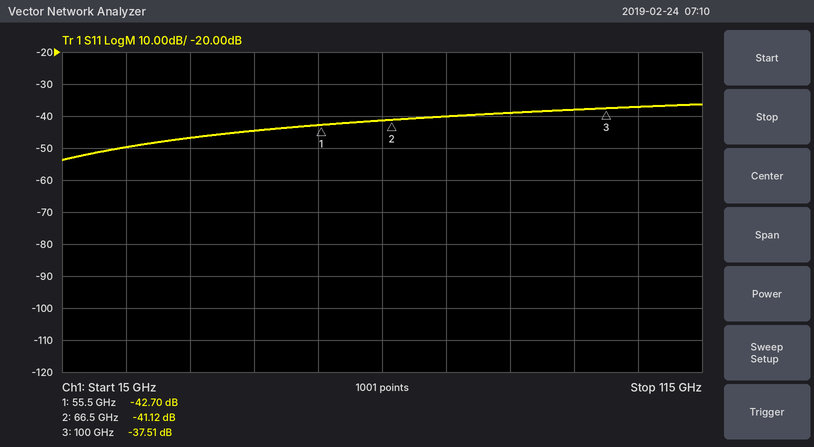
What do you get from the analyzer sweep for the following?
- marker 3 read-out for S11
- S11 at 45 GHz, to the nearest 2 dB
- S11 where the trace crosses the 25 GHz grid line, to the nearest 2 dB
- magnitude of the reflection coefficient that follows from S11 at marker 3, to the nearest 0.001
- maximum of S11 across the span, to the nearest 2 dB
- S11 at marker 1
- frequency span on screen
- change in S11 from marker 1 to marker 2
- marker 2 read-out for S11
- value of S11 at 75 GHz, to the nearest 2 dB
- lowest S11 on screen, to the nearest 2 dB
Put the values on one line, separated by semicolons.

-37.51 dB; -44 dB; -50 dB; 0.013; -36 dB; -42.70 dB; 100 GHz; 1.58 dB; -41.12 dB; -40 dB; -54 dB
